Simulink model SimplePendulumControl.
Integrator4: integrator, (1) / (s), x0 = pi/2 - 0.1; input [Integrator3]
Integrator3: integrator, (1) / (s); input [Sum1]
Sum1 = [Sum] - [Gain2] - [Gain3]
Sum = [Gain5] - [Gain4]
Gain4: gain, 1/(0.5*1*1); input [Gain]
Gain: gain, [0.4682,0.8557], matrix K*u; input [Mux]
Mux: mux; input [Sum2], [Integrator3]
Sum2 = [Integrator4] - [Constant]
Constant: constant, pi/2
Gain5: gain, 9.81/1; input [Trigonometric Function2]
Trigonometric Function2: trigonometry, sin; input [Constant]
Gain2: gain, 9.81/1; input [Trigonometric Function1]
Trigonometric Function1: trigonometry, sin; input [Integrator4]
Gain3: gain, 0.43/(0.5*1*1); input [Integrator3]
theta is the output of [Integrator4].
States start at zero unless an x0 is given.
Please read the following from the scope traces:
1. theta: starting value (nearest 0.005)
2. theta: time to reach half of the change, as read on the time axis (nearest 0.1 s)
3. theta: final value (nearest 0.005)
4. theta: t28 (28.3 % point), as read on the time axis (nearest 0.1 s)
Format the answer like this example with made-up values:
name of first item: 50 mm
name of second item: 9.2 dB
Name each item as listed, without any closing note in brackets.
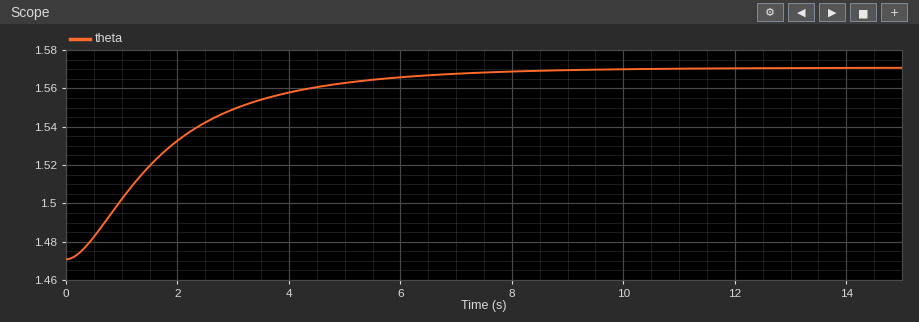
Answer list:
theta: starting value: 1.470
theta: time to reach half of the change, as read on the time axis: 1.5 s
theta: final value: 1.570
theta: t28 (28.3 % point), as read on the time axis: 0.9 s
